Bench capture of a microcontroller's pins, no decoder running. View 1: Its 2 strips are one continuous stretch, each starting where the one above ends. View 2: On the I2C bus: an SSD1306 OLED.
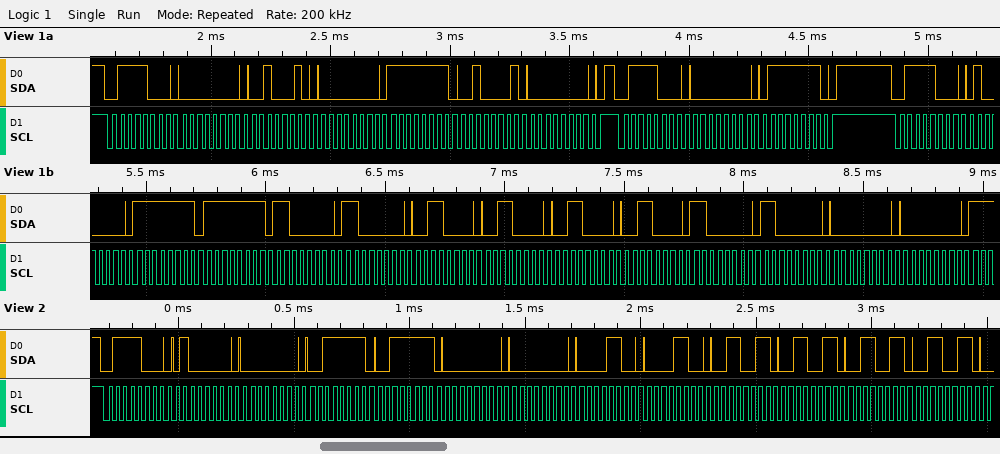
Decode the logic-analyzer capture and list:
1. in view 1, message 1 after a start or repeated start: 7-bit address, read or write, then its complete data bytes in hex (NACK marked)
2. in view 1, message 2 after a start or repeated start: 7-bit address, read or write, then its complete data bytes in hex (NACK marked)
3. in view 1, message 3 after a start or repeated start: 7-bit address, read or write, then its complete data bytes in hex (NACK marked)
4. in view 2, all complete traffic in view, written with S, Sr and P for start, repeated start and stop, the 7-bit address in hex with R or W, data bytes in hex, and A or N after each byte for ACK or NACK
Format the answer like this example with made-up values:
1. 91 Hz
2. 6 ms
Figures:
1. 0x3C write: 00 22 00 FF 21 00
2. 0x3C write: 00 7F
3. 0x3C write: 40 FF FF C0 C0 30 30 30 30 C0 C0 00 00
4. S 3CW A 40 A 00 A 3F A 3F A 00 A 00 A 0C A 0C A 33 A 33 A 33 A 33 A
